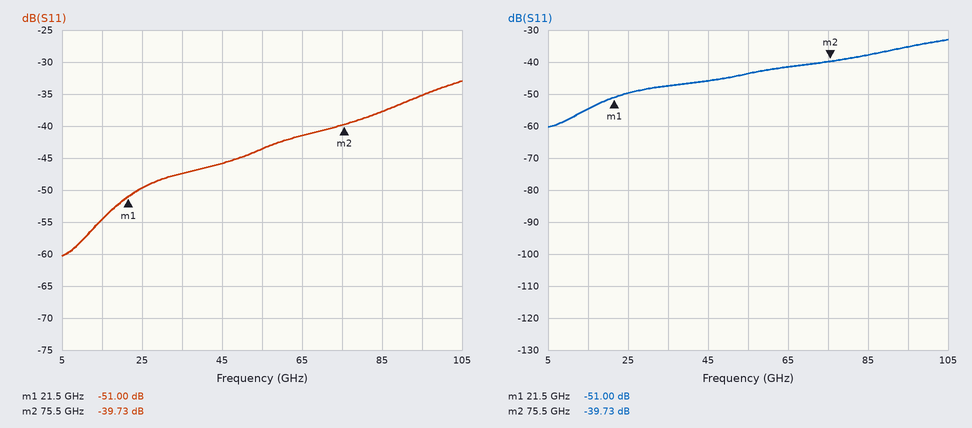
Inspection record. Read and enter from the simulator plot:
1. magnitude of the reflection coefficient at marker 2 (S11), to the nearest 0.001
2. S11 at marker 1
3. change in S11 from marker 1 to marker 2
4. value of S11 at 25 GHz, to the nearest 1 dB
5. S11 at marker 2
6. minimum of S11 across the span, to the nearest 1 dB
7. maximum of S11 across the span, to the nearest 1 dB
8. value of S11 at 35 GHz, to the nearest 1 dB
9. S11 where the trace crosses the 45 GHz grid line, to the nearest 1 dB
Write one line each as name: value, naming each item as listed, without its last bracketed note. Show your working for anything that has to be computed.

magnitude of the reflection coefficient at marker 2 (S11), to the nearest 0.001: 10^(-39.73/20) ≈ 0.010
S11 at marker 1: -51.00 dB
change in S11 from marker 1 to marker 2: -39.73 − (-51) = 11.27 dB
value of S11 at 25 GHz, to the nearest 1 dB: -50 dB
S11 at marker 2: -39.73 dB
minimum of S11 across the span, to the nearest 1 dB: -60 dB
maximum of S11 across the span, to the nearest 1 dB: -33 dB
value of S11 at 35 GHz, to the nearest 1 dB: -47 dB
S11 where the trace crosses the 45 GHz grid line, to the nearest 1 dB: -46 dB
